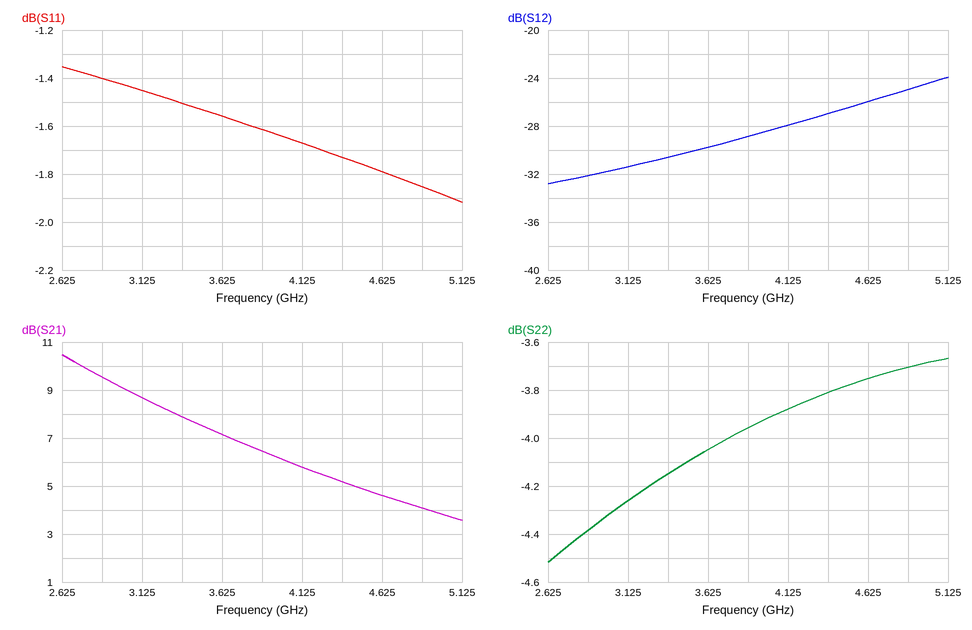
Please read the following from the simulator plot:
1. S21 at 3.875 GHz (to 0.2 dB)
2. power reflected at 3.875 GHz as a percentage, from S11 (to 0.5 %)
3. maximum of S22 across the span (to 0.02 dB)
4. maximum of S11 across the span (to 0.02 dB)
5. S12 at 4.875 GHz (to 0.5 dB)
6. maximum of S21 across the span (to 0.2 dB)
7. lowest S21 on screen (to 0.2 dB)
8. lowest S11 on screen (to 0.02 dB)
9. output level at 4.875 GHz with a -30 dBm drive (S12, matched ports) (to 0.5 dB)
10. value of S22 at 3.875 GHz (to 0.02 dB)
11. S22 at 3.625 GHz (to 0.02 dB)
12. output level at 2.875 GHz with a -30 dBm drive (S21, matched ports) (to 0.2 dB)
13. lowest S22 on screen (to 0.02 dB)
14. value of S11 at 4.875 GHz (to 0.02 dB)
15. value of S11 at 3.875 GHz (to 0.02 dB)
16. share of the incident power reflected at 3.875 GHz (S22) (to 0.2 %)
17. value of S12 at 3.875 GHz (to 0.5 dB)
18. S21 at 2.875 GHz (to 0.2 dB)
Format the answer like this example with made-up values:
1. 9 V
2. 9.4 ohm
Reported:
1. 6.4 dB
2. 69.0 %
3. -3.66 dB
4. -1.36 dB
5. -25.0 dB
6. 10.4 dB
7. 3.6 dB
8. -1.92 dB
9. -55.0 dBm
10. -3.96 dB
11. -4.04 dB
12. -20.4 dBm
13. -4.52 dB
14. -1.86 dB
15. -1.62 dB
16. 40.2 %
17. -29.0 dB
18. 9.6 dB
